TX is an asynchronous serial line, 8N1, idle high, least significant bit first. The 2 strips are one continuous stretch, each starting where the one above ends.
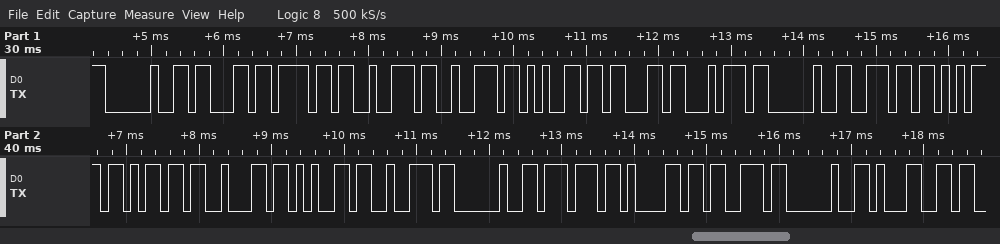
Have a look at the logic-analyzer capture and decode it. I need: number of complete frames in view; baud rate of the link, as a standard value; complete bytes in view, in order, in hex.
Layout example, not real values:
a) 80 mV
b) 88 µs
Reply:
a) 21
b) 9600 baud
c) 0x20 0x63 0x6F 0x72 0x72 0x65 0x63 0x74 0x20 0x6E 0x75 0x6D 0x62 0x65 0x72 0x20 0x77 0x61 0x73 0x20 0x31
